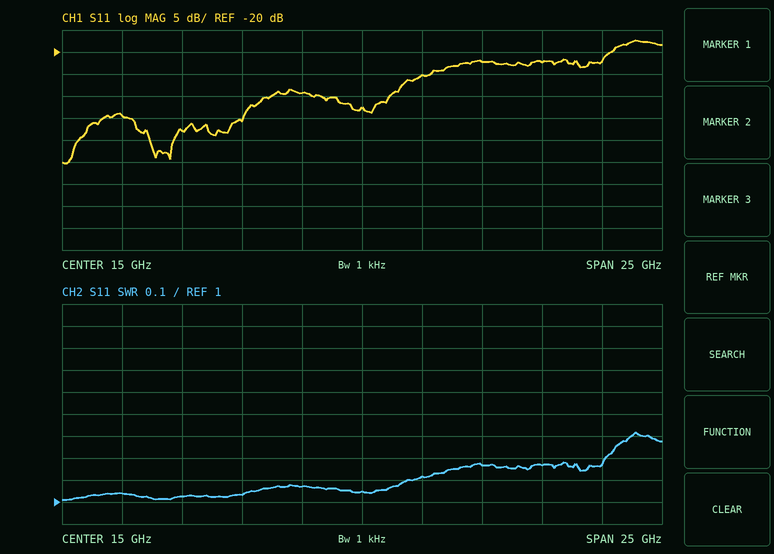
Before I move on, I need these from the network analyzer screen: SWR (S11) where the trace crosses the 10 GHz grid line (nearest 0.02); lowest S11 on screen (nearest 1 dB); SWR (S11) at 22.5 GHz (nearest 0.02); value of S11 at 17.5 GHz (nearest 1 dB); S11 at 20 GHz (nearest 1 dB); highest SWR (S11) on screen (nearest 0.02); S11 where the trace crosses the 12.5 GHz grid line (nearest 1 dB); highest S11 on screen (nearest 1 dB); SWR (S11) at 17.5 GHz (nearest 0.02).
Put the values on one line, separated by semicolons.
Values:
1.04; -45 dB; 1.16; -25 dB; -22 dB; 1.32; -29 dB; -17 dB; 1.12
